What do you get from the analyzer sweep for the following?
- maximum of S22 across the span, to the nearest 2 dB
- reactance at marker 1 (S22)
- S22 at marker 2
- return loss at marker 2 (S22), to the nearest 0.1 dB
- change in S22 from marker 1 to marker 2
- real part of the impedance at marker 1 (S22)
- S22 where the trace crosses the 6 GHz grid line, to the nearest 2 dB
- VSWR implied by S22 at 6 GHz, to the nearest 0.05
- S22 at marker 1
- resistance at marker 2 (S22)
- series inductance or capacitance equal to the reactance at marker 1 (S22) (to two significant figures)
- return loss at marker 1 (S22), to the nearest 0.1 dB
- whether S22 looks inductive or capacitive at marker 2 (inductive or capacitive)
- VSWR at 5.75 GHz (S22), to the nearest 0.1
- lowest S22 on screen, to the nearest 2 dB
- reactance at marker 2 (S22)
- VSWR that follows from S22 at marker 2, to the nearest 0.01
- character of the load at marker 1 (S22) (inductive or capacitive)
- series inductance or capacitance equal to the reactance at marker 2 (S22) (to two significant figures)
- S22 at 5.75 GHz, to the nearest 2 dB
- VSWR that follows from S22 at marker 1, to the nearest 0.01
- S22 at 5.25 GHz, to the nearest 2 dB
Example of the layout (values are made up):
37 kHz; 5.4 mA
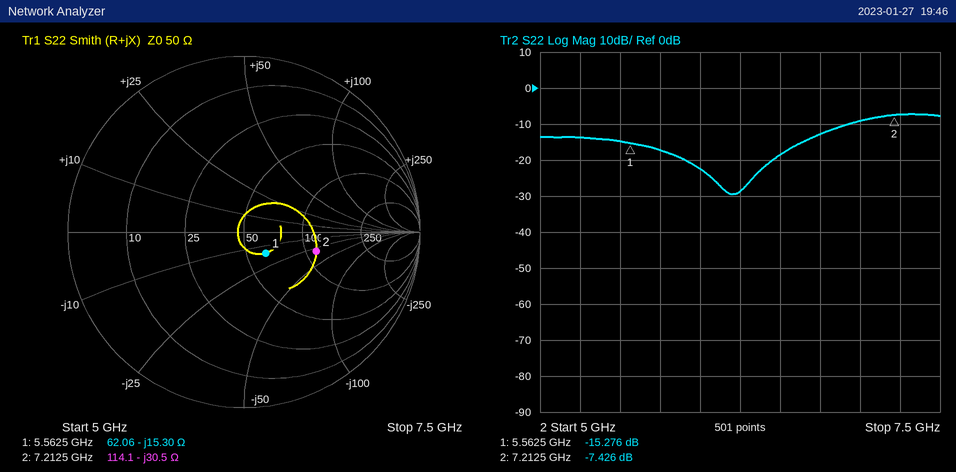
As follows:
-8 dB; -15.30 Ω; -7.426 dB; 7.4 dB; 7.850 dB; 62.06 Ω; -22 dB; 1.15; -15.276 dB; 114.1 Ω; 1.9 pF; 15.3 dB; capacitive; 1.3; -30 dB; -30.5 Ω; 2.48; capacitive; 720 fF; -18 dB; 1.42; -14 dB
